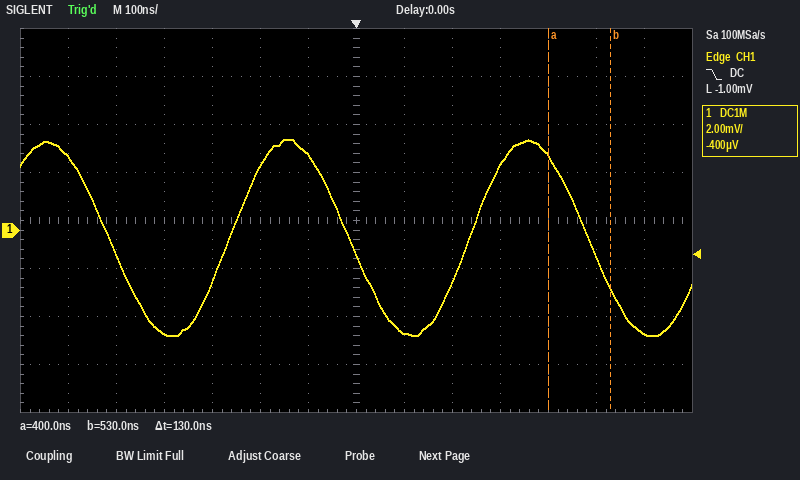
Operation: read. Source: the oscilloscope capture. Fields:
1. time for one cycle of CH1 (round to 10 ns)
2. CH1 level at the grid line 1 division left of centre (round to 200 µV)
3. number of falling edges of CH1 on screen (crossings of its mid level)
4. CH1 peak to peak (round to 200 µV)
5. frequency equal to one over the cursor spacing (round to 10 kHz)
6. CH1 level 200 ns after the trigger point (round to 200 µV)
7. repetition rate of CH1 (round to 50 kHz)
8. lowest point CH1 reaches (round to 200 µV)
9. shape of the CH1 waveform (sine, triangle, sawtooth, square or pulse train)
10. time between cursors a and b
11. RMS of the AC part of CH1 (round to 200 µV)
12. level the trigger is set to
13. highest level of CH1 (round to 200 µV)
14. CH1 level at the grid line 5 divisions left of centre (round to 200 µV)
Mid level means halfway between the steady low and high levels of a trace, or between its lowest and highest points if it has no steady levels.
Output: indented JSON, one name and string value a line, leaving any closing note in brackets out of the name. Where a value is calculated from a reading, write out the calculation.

{
  "time for one cycle of CH1": "500 ns",
  "CH1 level at the grid line 1 division left of centre": "3.2 mV",
  "number of falling edges of CH1 on screen": "3",
  "CH1 peak to peak": "3.8 mV − (-4.4 mV) = 8.2 mV",
  "frequency equal to one over the cursor spacing": "1 / 130 ns ≈ 7.69 MHz",
  "CH1 level 200 ns after the trigger point": "-2.2 mV",
  "repetition rate of CH1": "1 / 500 ns ≈ 2.00 MHz",
  "lowest point CH1 reaches": "-4.4 mV",
  "shape of the CH1 waveform": "sine",
  "time between cursors a and b": "130 ns",
  "RMS of the AC part of CH1": "8.2 mV / (2√2) ≈ 2.90 mV, so 2.8 mV to the nearest 200 µV",
  "level the trigger is set to": "-1.00 mV",
  "highest level of CH1": "3.8 mV",
  "CH1 level at the grid line 5 divisions left of centre": "-1.0 mV"
}
